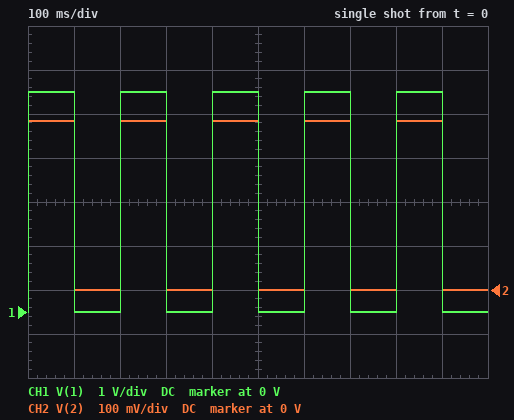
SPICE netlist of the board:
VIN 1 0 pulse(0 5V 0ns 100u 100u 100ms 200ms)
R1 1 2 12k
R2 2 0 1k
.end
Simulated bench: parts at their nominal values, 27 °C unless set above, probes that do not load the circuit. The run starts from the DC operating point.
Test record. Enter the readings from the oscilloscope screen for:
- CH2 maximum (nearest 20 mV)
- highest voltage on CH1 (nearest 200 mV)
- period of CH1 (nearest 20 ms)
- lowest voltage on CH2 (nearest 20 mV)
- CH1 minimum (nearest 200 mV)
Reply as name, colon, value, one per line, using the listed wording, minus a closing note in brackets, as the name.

CH2 maximum: 380 mV
highest voltage on CH1: 5.0 V
period of CH1: 200 ms
lowest voltage on CH2: 0 V
CH1 minimum: 0 V
